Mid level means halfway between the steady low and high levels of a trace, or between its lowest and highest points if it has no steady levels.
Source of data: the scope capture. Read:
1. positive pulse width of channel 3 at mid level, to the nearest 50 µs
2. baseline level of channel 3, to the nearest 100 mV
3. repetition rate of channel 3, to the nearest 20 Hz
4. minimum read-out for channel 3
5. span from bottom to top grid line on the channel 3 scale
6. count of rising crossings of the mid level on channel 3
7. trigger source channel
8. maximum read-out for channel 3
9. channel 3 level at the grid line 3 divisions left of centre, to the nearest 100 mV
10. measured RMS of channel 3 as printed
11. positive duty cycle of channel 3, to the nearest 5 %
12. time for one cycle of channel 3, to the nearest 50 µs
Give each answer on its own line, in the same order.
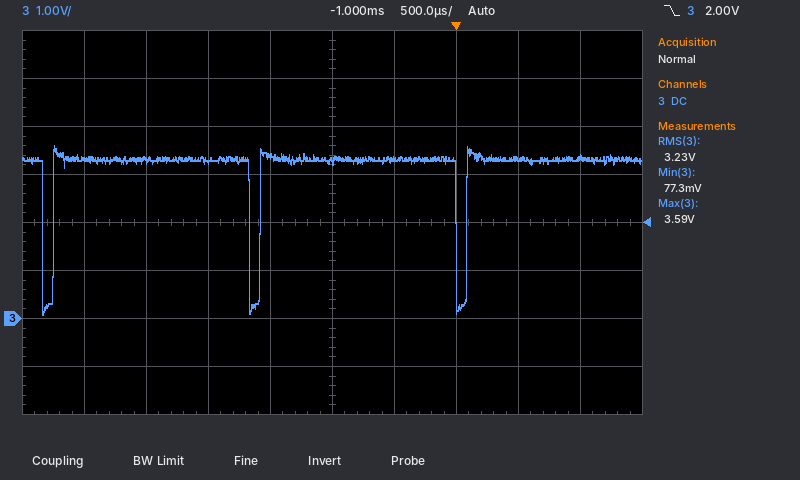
1.60 ms
3.3 V
600 Hz
77.3 mV
8 V
3
channel 3
3.59 V
3.3 V
3.23 V
95 %
1.65 ms
